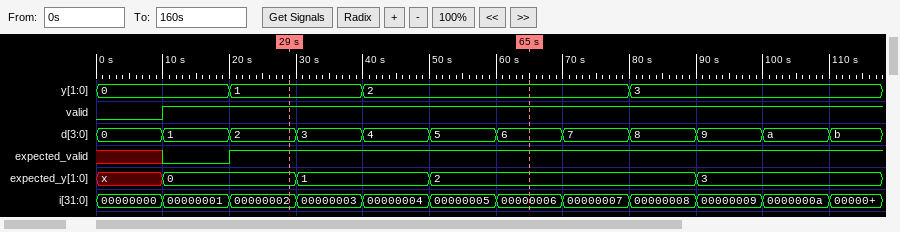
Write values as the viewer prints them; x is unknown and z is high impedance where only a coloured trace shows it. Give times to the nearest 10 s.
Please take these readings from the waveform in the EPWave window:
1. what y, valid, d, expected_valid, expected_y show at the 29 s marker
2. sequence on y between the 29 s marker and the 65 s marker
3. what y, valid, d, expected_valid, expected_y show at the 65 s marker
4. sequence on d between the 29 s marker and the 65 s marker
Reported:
y=1, valid=1, d=2, expected_valid=1, expected_y=0
1, 2
y=2, valid=1, d=6, expected_valid=1, expected_y=2
2, 3, 4, 5, 6
